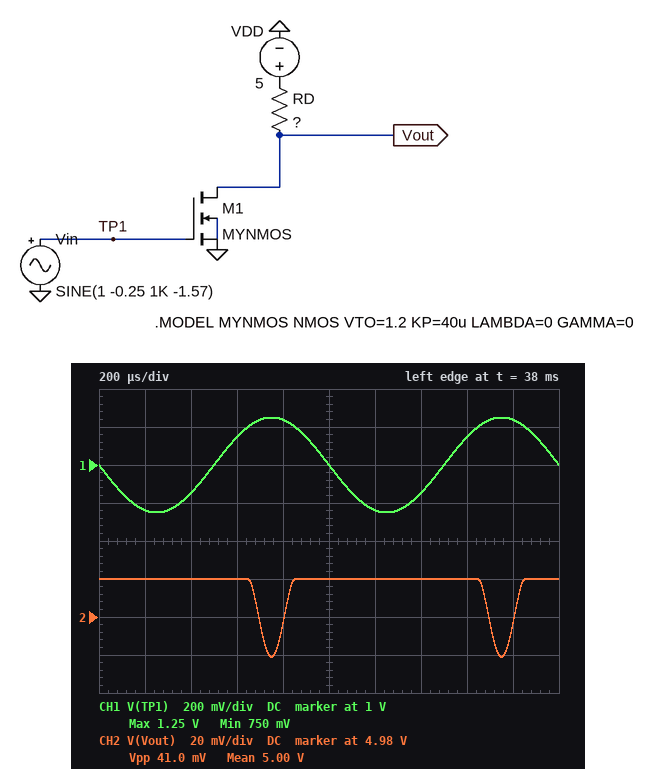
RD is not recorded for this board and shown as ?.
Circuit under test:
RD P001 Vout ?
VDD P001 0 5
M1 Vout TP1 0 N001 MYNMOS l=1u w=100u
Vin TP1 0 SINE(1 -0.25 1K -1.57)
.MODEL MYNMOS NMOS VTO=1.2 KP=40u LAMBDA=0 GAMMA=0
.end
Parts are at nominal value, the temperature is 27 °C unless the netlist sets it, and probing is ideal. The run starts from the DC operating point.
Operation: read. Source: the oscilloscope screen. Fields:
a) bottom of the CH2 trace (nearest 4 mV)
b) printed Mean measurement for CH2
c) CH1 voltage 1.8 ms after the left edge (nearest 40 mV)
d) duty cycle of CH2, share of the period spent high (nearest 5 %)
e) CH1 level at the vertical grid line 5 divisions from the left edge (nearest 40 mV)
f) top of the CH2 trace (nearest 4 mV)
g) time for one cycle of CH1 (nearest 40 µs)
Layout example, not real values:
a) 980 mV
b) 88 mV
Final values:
a) 4.960 V
b) 5.00 V
c) 1.24 V
d) 90 %
e) 1.00 V
f) 5.000 V
g) 1.00 ms
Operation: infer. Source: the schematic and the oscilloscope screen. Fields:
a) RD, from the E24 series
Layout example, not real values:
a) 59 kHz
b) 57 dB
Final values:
a) 8.2 kΩ
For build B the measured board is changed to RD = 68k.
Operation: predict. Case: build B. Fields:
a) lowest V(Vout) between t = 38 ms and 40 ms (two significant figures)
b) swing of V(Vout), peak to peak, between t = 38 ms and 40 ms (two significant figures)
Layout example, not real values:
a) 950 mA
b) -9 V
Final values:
a) 4.7 V
b) 340 mV
